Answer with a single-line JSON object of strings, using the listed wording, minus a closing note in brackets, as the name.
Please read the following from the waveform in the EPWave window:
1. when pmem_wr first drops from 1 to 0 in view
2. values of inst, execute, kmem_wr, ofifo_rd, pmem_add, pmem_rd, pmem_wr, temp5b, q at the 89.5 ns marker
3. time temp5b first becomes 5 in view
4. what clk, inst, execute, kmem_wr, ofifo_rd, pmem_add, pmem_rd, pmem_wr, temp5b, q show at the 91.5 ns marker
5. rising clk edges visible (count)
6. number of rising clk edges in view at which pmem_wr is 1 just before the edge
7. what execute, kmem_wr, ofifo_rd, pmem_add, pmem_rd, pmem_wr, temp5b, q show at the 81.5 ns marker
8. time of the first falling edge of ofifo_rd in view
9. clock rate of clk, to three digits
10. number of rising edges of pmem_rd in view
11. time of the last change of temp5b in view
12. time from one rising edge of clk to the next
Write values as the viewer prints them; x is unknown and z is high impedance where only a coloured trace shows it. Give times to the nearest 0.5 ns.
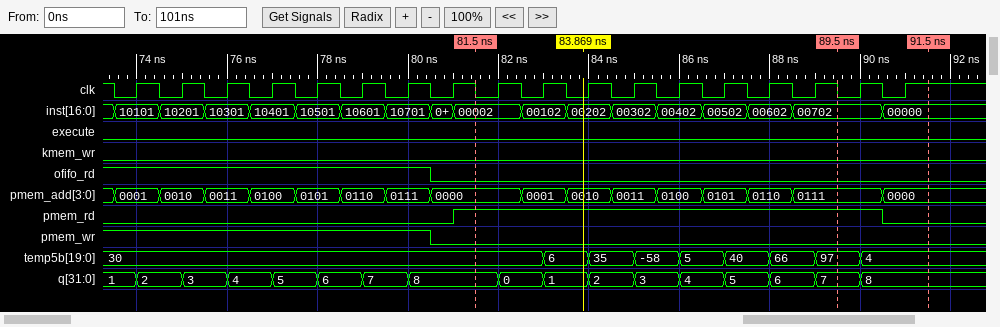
{"when pmem_wr first drops from 1 to 0 in view": "80.5 ns", "values of inst, execute, kmem_wr, ofifo_rd, pmem_add, pmem_rd, pmem_wr, temp5b, q at the 89.5 ns marker": "inst=00702, execute=0, kmem_wr=0, ofifo_rd=0, pmem_add=0111, pmem_rd=1, pmem_wr=0, temp5b=97, q=7", "time temp5b first becomes 5 in view": "86 ns", "what clk, inst, execute, kmem_wr, ofifo_rd, pmem_add, pmem_rd, pmem_wr, temp5b, q show at the 91.5 ns marker": "clk=1, inst=00000, execute=0, kmem_wr=0, ofifo_rd=0, pmem_add=0000, pmem_rd=0, pmem_wr=0, temp5b=4, q=8", "rising clk edges visible": "18", "number of rising clk edges in view at which pmem_wr is 1 just before the edge": "7", "what execute, kmem_wr, ofifo_rd, pmem_add, pmem_rd, pmem_wr, temp5b, q show at the 81.5 ns marker": "execute=0, kmem_wr=0, ofifo_rd=0, pmem_add=0000, pmem_rd=1, pmem_wr=0, temp5b=30, q=8", "time of the first falling edge of ofifo_rd in view": "80.5 ns", "clock rate of clk, to three digits": "1.00 GHz", "number of rising edges of pmem_rd in view": "1", "time of the last change of temp5b in view": "90 ns", "time from one rising edge of clk to the next": "1 ns"}
